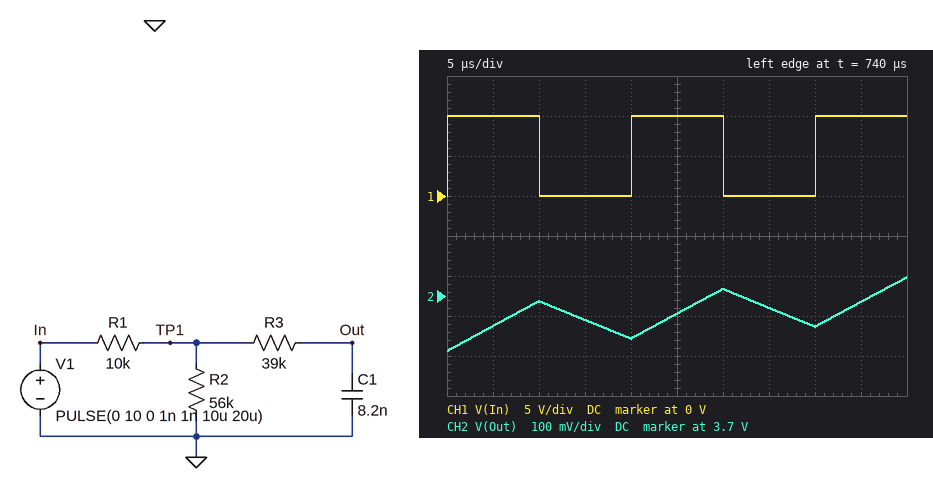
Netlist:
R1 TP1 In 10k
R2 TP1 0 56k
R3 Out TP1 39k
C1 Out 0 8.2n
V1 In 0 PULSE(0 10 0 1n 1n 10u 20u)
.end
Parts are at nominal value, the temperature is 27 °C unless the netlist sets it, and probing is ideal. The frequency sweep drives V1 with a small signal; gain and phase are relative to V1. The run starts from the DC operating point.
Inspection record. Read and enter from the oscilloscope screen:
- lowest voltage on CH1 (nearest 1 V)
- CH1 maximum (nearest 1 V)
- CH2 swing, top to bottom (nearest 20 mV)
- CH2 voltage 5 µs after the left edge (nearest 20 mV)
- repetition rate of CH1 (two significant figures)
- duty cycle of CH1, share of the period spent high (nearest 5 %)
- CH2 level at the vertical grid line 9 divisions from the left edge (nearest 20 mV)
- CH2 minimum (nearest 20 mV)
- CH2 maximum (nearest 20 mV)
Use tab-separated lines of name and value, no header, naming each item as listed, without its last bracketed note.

lowest voltage on CH1	0 V
CH1 maximum	10 V
CH2 swing, top to bottom	180 mV
CH2 voltage 5 µs after the left edge	3.62 V
repetition rate of CH1	50 kHz
duty cycle of CH1, share of the period spent high	50 %
CH2 level at the vertical grid line 9 divisions from the left edge	3.68 V
CH2 minimum	3.56 V
CH2 maximum	3.74 V
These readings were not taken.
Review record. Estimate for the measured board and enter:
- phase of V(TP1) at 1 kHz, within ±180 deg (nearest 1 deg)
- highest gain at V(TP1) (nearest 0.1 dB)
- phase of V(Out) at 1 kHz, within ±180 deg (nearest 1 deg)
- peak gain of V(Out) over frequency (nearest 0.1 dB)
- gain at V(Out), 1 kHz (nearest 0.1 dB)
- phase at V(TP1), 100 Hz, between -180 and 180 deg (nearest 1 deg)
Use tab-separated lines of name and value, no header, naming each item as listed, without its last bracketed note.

phase of V(TP1) at 1 kHz, within ±180 deg	-4 deg
highest gain at V(TP1)	-1.4 dB
phase of V(Out) at 1 kHz, within ±180 deg	-68 deg
peak gain of V(Out) over frequency	-1.4 dB
gain at V(Out), 1 kHz	-9.9 dB
phase at V(TP1), 100 Hz, between -180 and 180 deg	-2 deg
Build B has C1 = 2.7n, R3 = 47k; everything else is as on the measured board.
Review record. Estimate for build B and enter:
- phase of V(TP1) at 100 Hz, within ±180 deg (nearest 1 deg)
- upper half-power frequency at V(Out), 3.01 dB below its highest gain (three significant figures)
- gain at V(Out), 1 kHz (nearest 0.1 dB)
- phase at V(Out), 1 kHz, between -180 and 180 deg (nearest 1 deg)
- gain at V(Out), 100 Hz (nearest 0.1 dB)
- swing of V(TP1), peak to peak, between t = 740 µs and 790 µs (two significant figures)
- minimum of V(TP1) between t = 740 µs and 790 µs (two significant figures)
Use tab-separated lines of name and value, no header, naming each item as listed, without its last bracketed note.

phase of V(TP1) at 100 Hz, within ±180 deg	-1 deg
upper half-power frequency at V(Out), 3.01 dB below its highest gain	1.06 kHz
gain at V(Out), 1 kHz	-4.2 dB
phase at V(Out), 1 kHz, between -180 and 180 deg	-43 deg
gain at V(Out), 100 Hz	-1.5 dB
swing of V(TP1), peak to peak, between t = 740 µs and 790 µs	7.2 V
minimum of V(TP1) between t = 740 µs and 790 µs	620 mV
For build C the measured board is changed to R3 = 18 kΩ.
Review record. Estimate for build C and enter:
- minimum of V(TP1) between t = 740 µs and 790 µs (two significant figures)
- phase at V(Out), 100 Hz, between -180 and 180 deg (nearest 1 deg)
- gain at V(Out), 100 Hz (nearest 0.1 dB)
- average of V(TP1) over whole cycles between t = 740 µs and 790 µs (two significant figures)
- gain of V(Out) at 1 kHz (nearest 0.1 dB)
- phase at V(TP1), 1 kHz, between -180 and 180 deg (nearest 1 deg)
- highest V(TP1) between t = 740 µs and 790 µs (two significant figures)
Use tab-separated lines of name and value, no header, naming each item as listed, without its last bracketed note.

minimum of V(TP1) between t = 740 µs and 790 µs	1.3 V
phase at V(Out), 100 Hz, between -180 and 180 deg	-8 deg
gain at V(Out), 100 Hz	-1.5 dB
average of V(TP1) over whole cycles between t = 740 µs and 790 µs	4.2 V
gain of V(Out) at 1 kHz	-6.0 dB
phase at V(TP1), 1 kHz, between -180 and 180 deg	-11 deg
highest V(TP1) between t = 740 µs and 790 µs	7.1 V
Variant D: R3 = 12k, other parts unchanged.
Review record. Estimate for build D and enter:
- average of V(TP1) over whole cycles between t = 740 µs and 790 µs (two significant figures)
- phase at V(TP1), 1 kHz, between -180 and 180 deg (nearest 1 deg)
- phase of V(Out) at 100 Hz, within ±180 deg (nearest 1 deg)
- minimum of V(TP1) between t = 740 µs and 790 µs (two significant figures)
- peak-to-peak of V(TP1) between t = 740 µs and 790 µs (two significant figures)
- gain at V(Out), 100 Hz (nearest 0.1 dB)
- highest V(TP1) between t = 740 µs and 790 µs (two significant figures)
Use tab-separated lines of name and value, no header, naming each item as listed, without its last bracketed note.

average of V(TP1) over whole cycles between t = 740 µs and 790 µs	4.2 V
phase at V(TP1), 1 kHz, between -180 and 180 deg	-15 deg
phase of V(Out) at 100 Hz, within ±180 deg	-6 deg
minimum of V(TP1) between t = 740 µs and 790 µs	1.7 V
peak-to-peak of V(TP1) between t = 740 µs and 790 µs	5.1 V
gain at V(Out), 100 Hz	-1.5 dB
highest V(TP1) between t = 740 µs and 790 µs	6.8 V
